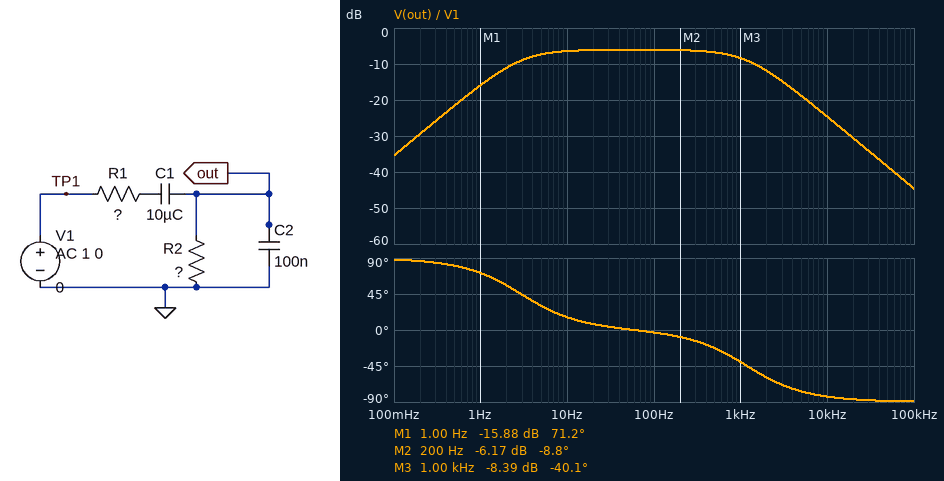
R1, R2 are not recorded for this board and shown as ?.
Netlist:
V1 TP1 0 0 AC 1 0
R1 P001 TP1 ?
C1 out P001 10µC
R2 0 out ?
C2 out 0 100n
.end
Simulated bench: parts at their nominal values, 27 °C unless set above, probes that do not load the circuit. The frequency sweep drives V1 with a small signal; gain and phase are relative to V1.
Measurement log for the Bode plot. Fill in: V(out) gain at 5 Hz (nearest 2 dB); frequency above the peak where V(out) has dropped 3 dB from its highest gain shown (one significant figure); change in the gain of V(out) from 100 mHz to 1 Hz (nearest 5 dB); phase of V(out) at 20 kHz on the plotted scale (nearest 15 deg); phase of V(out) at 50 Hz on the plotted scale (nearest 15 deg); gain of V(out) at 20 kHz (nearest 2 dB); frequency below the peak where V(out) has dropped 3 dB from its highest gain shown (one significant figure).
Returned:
-8 dB
1 kHz
20 dB
-90 deg
0 deg
-30 dB
3 Hz
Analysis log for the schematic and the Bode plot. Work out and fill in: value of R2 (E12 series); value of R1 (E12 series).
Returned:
2.7 kΩ
2.7 kΩ
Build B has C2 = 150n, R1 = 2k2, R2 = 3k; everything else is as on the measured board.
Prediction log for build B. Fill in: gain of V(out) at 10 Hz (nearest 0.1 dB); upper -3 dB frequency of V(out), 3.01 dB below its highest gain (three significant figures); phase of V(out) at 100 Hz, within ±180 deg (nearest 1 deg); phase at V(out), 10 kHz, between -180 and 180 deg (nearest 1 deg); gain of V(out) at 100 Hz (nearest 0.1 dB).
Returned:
-5.2 dB
846 Hz
-5 deg
-85 deg
-4.9 dB
